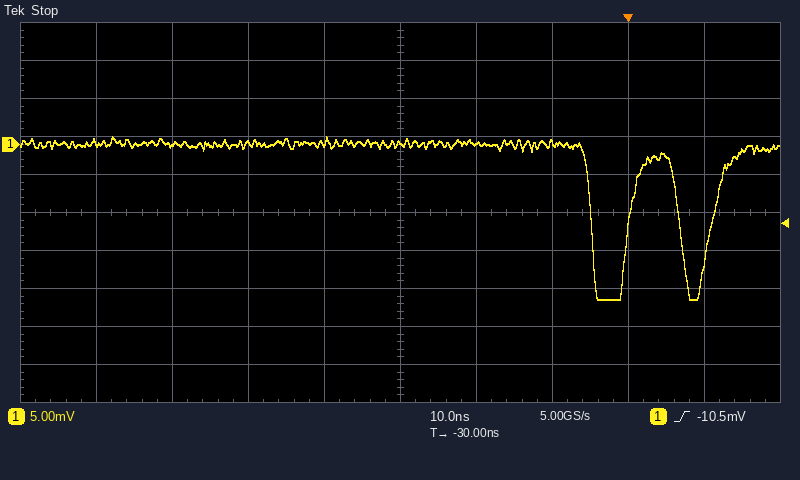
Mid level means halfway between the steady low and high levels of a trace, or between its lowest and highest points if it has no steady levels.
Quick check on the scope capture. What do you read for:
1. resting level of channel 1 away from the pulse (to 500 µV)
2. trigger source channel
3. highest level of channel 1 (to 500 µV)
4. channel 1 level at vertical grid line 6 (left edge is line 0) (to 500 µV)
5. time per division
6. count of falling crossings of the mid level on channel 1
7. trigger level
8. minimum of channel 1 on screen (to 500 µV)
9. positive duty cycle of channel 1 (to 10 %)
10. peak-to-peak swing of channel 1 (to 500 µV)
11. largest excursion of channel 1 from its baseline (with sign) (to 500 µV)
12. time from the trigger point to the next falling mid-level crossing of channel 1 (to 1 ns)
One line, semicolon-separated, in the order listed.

0.0 mV; channel 1; 1.0 mV; 0.0 mV; 10 ns; 2; -10.5 mV; -20.5 mV; 60 %; 21.5 mV; -20.5 mV; 7 ns
